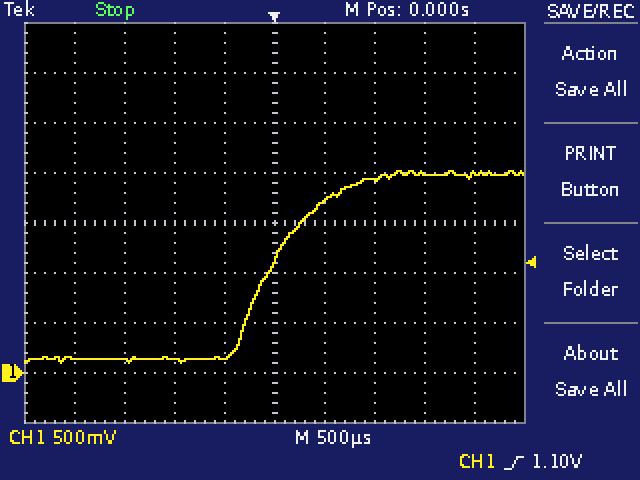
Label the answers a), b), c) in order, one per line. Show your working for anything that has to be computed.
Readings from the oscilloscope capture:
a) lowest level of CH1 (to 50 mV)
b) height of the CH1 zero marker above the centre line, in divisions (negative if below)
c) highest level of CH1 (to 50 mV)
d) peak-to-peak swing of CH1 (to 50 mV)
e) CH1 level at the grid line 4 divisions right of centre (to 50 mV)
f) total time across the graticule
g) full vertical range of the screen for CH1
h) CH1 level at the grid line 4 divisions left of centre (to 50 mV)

a) 100 mV
b) -3.0 div
c) 2.00 V
d) 2.00 V − (100 mV) = 1.90 V
e) 2.00 V
f) 5 ms
g) 4 V
h) 150 mV
